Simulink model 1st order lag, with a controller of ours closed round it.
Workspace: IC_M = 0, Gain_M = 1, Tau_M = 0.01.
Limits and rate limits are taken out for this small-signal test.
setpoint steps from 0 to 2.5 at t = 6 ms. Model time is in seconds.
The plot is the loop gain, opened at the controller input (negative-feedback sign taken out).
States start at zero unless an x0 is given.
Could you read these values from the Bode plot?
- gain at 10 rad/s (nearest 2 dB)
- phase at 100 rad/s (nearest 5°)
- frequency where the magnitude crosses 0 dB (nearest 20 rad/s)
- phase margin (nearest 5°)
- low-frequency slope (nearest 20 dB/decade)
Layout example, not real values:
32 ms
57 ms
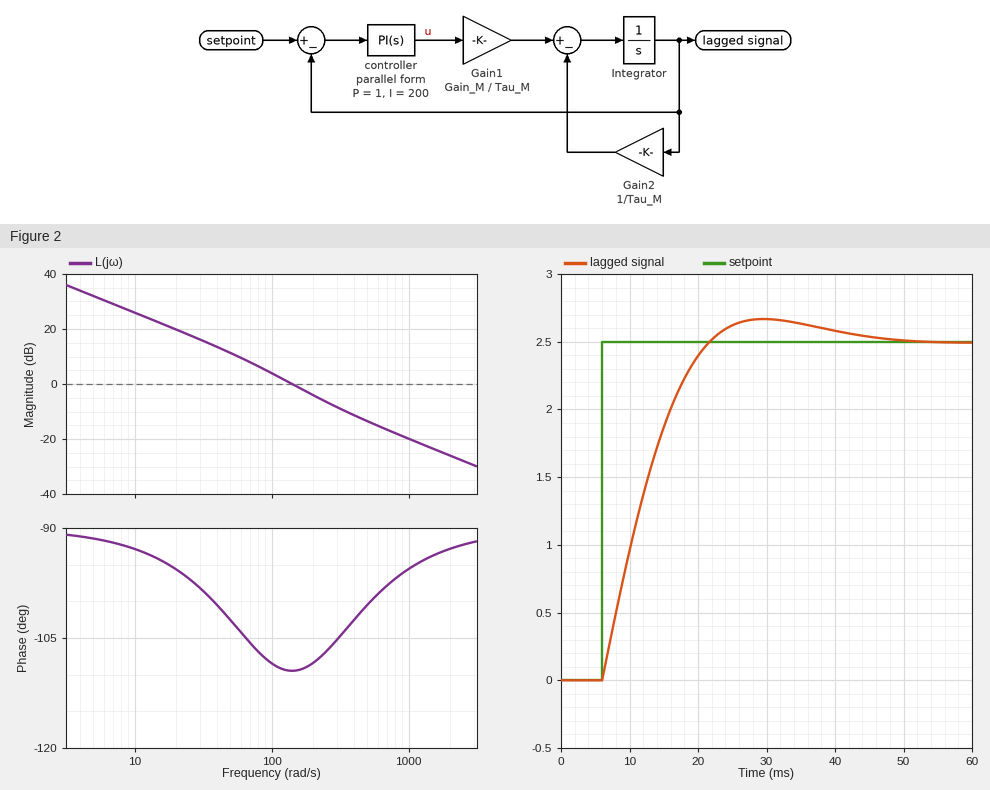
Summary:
26 dB
-110°
140 rad/s
70°
-20 dB/decade
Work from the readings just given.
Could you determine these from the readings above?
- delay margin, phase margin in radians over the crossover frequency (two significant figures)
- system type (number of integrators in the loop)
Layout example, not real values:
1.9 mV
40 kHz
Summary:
0.0087 s
1
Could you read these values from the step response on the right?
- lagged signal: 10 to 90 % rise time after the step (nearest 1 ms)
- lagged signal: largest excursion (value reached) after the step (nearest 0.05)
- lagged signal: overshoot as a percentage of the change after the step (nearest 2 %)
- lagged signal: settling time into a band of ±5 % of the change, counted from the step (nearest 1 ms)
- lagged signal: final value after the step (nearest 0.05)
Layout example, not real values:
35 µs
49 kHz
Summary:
11 ms
2.65
6 %
30 ms
2.50
